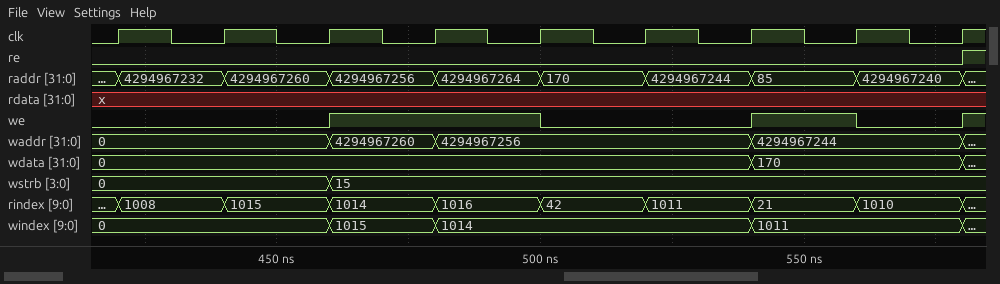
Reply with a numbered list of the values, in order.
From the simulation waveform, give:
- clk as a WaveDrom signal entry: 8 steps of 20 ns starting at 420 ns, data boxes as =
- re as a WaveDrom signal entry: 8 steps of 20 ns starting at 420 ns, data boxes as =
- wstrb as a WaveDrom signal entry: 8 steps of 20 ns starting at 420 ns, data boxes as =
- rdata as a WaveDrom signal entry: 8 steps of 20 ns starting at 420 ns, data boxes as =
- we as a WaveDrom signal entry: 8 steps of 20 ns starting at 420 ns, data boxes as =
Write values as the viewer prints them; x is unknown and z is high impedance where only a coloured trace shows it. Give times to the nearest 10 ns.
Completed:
1. {name: 'clk', wave: 'p.......'}
2. {name: 're', wave: '0.......'}
3. {name: 'wstrb', wave: '=.=.....', data: '0 15'}
4. {name: 'rdata', wave: 'x.......'}
5. {name: 'we', wave: '0.1.0.10'}
